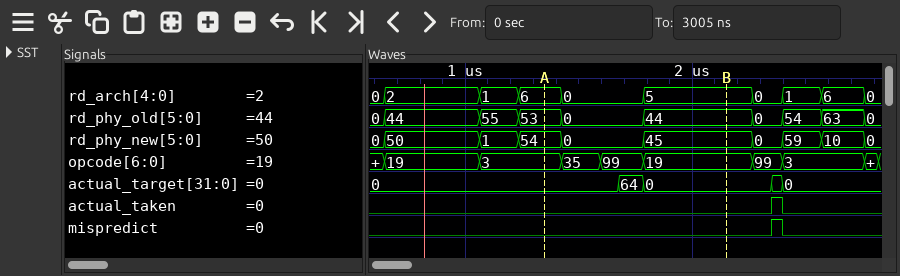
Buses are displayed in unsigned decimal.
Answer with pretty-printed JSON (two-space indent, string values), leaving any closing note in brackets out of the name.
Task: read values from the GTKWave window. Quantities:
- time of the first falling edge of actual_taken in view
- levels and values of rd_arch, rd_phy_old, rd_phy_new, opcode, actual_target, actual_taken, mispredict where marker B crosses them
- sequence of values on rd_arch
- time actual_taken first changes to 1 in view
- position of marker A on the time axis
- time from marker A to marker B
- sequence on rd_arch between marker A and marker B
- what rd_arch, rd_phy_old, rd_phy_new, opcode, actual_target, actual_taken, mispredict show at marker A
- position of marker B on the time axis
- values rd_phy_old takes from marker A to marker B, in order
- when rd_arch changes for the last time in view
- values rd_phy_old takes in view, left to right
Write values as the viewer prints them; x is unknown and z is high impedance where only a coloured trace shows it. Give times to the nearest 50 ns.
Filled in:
{
  "time of the first falling edge of actual_taken in view": "2400 ns",
  "levels and values of rd_arch, rd_phy_old, rd_phy_new, opcode, actual_target, actual_taken, mispredict where marker B crosses them": "rd_arch=5, rd_phy_old=44, rd_phy_new=45, opcode=19, actual_target=0, actual_taken=0, mispredict=0",
  "sequence of values on rd_arch": "0, 2, 1, 6, 0, 5, 0, 1, 6, 0",
  "time actual_taken first changes to 1 in view": "2350 ns",
  "position of marker A on the time axis": "1350 ns",
  "time from marker A to marker B": "800 ns",
  "sequence on rd_arch between marker A and marker B": "6, 0, 5",
  "what rd_arch, rd_phy_old, rd_phy_new, opcode, actual_target, actual_taken, mispredict show at marker A": "rd_arch=6, rd_phy_old=53, rd_phy_new=54, opcode=3, actual_target=0, actual_taken=0, mispredict=0",
  "position of marker B on the time axis": "2150 ns",
  "values rd_phy_old takes from marker A to marker B, in order": "53, 0, 44",
  "when rd_arch changes for the last time in view": "2750 ns",
  "values rd_phy_old takes in view, left to right": "0, 44, 55, 53, 0, 44, 0, 54, 63, 0"
}
